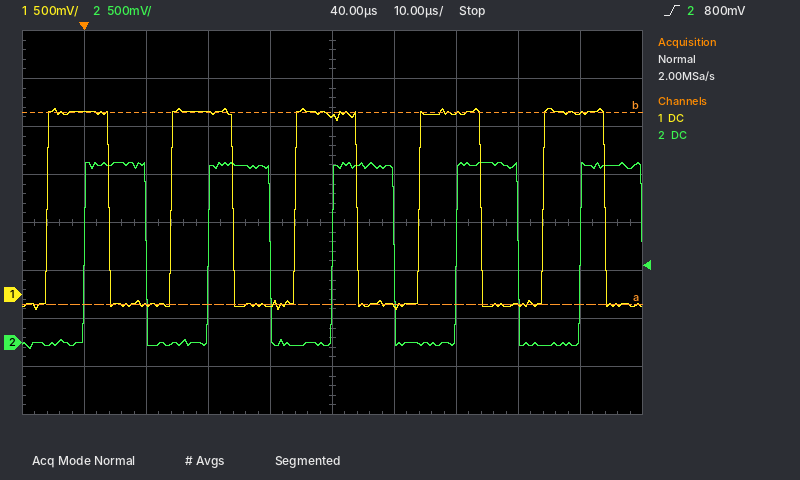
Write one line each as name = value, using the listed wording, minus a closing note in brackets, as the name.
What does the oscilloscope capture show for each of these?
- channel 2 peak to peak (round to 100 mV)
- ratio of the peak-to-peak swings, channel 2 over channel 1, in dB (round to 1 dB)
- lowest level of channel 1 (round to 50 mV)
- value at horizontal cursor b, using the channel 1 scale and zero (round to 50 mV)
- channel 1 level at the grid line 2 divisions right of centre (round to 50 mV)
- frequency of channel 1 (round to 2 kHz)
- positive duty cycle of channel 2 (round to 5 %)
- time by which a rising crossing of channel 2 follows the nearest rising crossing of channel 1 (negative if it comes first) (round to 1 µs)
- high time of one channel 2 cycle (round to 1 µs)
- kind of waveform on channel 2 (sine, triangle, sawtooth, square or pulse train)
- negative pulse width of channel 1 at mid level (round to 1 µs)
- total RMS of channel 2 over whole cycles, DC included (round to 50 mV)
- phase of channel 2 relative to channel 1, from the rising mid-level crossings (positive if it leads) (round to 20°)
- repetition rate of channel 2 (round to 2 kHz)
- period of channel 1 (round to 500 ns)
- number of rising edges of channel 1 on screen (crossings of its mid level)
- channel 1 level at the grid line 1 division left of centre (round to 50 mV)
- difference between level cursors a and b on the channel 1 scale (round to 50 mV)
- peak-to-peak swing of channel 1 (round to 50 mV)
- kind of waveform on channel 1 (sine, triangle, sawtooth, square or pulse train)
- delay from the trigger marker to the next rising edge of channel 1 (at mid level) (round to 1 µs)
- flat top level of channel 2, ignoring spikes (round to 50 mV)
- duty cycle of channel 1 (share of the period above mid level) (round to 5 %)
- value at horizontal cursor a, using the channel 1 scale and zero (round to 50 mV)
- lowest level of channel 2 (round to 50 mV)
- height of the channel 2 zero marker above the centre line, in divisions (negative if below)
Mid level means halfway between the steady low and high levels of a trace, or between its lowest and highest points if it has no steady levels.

channel 2 peak to peak = 1.90 V
ratio of the peak-to-peak swings, channel 2 over channel 1, in dB = -1 dB
lowest level of channel 1 = -150 mV
value at horizontal cursor b, using the channel 1 scale and zero = 1.90 V
channel 1 level at the grid line 2 divisions right of centre = 1.90 V
frequency of channel 1 = 50 kHz
positive duty cycle of channel 2 = 50 %
time by which a rising crossing of channel 2 follows the nearest rising crossing of channel 1 (negative if it comes first) = +6 µs
high time of one channel 2 cycle = 10 µs
kind of waveform on channel 2 = square
negative pulse width of channel 1 at mid level = 10 µs
total RMS of channel 2 over whole cycles, DC included = 1.30 V
phase of channel 2 relative to channel 1, from the rising mid-level crossings (positive if it leads) = -100°
repetition rate of channel 2 = 50 kHz
period of channel 1 = 20.0 µs
number of rising edges of channel 1 on screen = 5
channel 1 level at the grid line 1 division left of centre = -100 mV
difference between level cursors a and b on the channel 1 scale = 2.00 V
peak-to-peak swing of channel 1 = 2.10 V
kind of waveform on channel 1 = square
delay from the trigger marker to the next rising edge of channel 1 (at mid level) = 14 µs
flat top level of channel 2, ignoring spikes = 1.85 V
duty cycle of channel 1 (share of the period above mid level) = 50 %
value at horizontal cursor a, using the channel 1 scale and zero = -100 mV
lowest level of channel 2 = -50 mV
height of the channel 2 zero marker above the centre line, in divisions = -2.5 div
